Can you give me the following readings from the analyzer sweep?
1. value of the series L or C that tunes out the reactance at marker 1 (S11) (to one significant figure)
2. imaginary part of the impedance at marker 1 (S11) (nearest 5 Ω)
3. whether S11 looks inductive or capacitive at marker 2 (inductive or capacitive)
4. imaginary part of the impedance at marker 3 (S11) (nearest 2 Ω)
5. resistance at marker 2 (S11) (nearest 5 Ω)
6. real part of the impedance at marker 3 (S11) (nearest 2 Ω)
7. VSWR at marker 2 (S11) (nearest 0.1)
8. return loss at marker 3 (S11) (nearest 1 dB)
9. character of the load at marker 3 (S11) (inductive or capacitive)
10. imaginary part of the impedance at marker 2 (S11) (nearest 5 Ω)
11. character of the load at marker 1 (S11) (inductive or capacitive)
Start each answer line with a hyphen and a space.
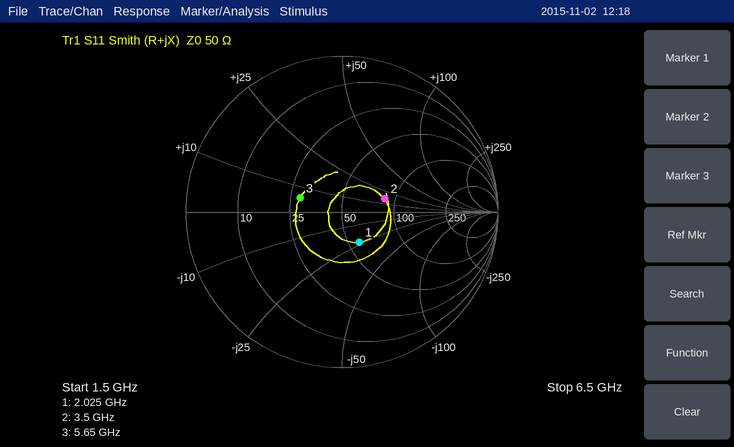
- 2 nH
- -25 Ω
- inductive
- +6 Ω
- 85 Ω
- 28 Ω
- 1.8
- 11 dB
- inductive
- +15 Ω
- capacitive
